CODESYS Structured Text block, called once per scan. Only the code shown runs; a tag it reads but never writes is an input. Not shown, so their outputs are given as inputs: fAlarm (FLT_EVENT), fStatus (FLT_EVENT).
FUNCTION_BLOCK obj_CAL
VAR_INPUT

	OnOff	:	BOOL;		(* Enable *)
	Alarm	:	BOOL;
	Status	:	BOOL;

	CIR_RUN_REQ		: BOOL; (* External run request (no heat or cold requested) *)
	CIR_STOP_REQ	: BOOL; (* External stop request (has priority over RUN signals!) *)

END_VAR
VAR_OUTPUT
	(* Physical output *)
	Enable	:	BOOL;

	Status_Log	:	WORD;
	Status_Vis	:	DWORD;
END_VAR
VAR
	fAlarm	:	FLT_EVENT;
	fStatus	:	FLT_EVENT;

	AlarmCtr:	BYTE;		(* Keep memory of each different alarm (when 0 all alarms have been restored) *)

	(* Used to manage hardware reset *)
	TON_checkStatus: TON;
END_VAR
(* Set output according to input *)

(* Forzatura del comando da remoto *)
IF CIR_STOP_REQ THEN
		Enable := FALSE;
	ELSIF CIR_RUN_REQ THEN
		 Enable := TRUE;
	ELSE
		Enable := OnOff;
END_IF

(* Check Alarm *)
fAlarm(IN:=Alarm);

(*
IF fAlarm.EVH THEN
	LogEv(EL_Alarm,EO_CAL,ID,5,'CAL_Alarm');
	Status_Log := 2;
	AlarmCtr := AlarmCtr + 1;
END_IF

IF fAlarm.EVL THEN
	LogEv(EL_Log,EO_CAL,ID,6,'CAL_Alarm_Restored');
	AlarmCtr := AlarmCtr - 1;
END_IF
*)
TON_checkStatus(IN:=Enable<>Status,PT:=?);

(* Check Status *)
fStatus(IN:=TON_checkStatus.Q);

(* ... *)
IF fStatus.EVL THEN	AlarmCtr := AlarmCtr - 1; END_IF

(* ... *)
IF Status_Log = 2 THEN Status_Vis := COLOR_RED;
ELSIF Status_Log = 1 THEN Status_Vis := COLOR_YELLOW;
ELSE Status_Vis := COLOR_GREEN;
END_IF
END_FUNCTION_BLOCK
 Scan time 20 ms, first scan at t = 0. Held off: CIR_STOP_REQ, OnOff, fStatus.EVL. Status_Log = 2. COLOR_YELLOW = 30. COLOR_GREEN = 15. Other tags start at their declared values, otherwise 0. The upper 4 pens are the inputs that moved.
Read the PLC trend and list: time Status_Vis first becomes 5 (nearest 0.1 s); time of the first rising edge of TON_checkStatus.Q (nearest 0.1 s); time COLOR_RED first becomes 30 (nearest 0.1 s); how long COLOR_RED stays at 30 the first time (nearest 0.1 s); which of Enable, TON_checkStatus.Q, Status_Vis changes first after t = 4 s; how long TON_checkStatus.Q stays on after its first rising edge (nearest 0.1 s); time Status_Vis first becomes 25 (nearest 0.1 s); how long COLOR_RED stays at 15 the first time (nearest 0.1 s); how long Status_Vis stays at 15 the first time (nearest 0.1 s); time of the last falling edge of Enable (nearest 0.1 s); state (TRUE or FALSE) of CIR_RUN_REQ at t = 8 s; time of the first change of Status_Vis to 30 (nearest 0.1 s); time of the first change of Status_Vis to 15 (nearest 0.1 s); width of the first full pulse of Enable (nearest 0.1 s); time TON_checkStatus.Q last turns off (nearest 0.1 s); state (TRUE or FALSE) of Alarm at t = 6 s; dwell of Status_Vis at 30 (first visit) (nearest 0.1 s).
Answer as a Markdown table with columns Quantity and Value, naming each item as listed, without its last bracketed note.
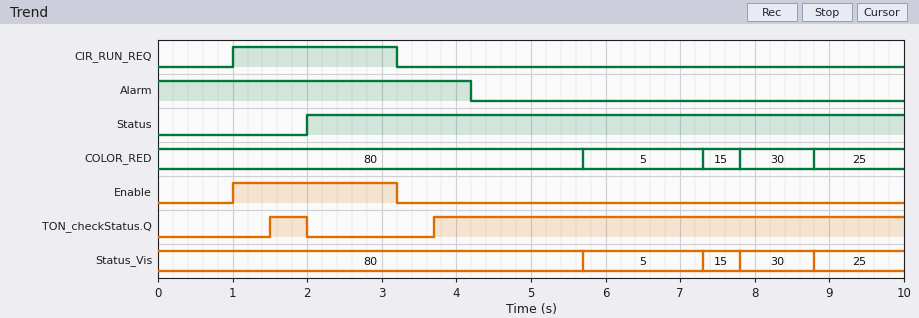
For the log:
| Quantity | Value |
|---|---|
| time Status_Vis first becomes 5 | 5.7 s |
| time of the first rising edge of TON_checkStatus.Q | 1.5 s |
| time COLOR_RED first becomes 30 | 7.8 s |
| how long COLOR_RED stays at 30 the first time | 1.0 s |
| which of Enable, TON_checkStatus.Q, Status_Vis changes first after t = 4 s | Status_Vis |
| how long TON_checkStatus.Q stays on after its first rising edge | 0.5 s |
| time Status_Vis first becomes 25 | 8.8 s |
| how long COLOR_RED stays at 15 the first time | 0.5 s |
| how long Status_Vis stays at 15 the first time | 0.5 s |
| time of the last falling edge of Enable | 3.2 s |
| state (TRUE or FALSE) of CIR_RUN_REQ at t = 8 s | FALSE |
| time of the first change of Status_Vis to 30 | 7.8 s |
| time of the first change of Status_Vis to 15 | 7.3 s |
| width of the first full pulse of Enable | 2.2 s |
| time TON_checkStatus.Q last turns off | 2.0 s |
| state (TRUE or FALSE) of Alarm at t = 6 s | FALSE |
| dwell of Status_Vis at 30 (first visit) | 1.0 s |
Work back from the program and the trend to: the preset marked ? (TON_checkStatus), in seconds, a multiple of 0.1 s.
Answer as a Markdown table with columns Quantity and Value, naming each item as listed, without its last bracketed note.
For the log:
| Quantity | Value |
|---|---|
| the preset marked ? (TON_checkStatus), in seconds, a multiple of 0.1 s | 0.5 s |
